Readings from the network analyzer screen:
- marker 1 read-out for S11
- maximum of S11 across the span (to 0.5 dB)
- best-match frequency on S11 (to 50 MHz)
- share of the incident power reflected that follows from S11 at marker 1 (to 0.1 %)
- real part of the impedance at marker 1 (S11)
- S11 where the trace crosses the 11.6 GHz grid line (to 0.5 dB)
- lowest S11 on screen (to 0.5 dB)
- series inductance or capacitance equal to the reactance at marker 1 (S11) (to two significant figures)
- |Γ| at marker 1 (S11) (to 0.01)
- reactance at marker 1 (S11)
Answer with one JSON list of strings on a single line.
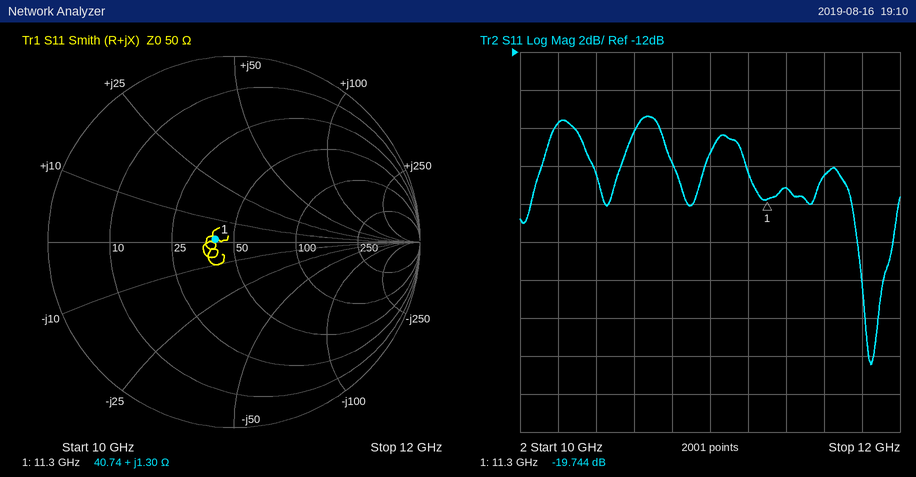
["-19.744 dB", "-15.5 dB", "11.85 GHz", "1.1 %", "40.74 Ω", "-18.5 dB", "-28.5 dB", "18 pH", "0.10", "+1.30 Ω"]
